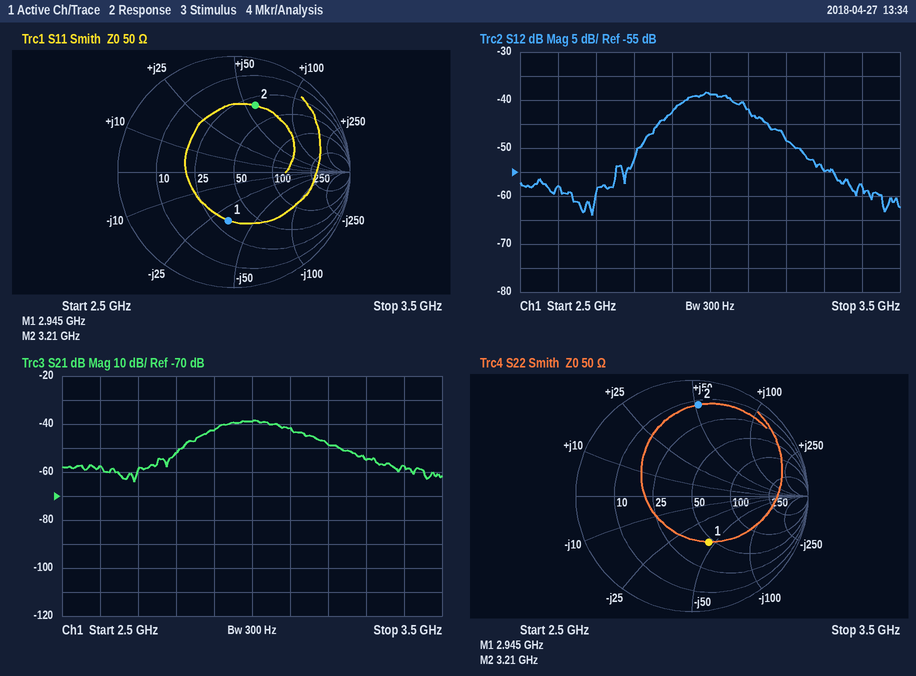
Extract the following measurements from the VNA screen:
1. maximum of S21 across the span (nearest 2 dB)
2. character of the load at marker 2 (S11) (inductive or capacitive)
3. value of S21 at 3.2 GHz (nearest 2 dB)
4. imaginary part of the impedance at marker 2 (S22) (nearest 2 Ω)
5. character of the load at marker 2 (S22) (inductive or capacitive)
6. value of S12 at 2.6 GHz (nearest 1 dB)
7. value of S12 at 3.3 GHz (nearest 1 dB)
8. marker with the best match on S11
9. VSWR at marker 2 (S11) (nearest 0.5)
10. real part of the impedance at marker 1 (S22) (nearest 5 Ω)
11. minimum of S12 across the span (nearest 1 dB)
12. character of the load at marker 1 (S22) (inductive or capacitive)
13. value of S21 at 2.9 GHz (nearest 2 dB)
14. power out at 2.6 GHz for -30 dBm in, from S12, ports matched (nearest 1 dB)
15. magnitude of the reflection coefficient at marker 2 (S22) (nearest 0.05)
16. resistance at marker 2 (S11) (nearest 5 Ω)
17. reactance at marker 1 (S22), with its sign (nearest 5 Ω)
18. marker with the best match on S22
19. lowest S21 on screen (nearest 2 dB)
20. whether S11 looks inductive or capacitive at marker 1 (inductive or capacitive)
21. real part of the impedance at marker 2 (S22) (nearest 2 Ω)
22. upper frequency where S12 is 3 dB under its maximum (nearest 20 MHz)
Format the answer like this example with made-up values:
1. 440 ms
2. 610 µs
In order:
1. -38 dB
2. inductive
3. -48 dB
4. +52 Ω
5. inductive
6. -58 dB
7. -55 dB
8. marker 1
9. 4.0
10. 45 Ω
11. -64 dB
12. capacitive
13. -42 dB
14. -88 dBm
15. 0.80
16. 30 Ω
17. -45 Ω
18. marker 1
19. -64 dB
20. capacitive
21. 12 Ω
22. 3.10 GHz
